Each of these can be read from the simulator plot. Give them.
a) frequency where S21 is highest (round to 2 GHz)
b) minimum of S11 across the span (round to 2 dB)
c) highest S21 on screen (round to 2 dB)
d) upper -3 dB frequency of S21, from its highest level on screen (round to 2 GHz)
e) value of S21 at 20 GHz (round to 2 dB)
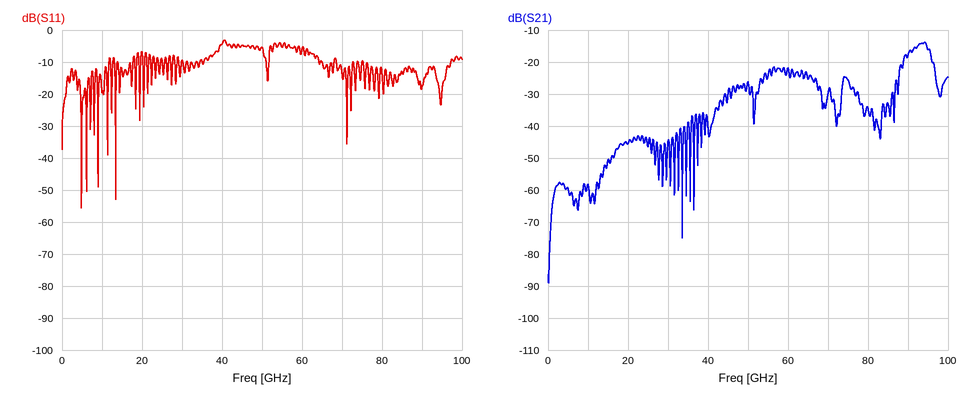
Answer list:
94 GHz
-56 dB
-14 dB
96 GHz
-46 dB
